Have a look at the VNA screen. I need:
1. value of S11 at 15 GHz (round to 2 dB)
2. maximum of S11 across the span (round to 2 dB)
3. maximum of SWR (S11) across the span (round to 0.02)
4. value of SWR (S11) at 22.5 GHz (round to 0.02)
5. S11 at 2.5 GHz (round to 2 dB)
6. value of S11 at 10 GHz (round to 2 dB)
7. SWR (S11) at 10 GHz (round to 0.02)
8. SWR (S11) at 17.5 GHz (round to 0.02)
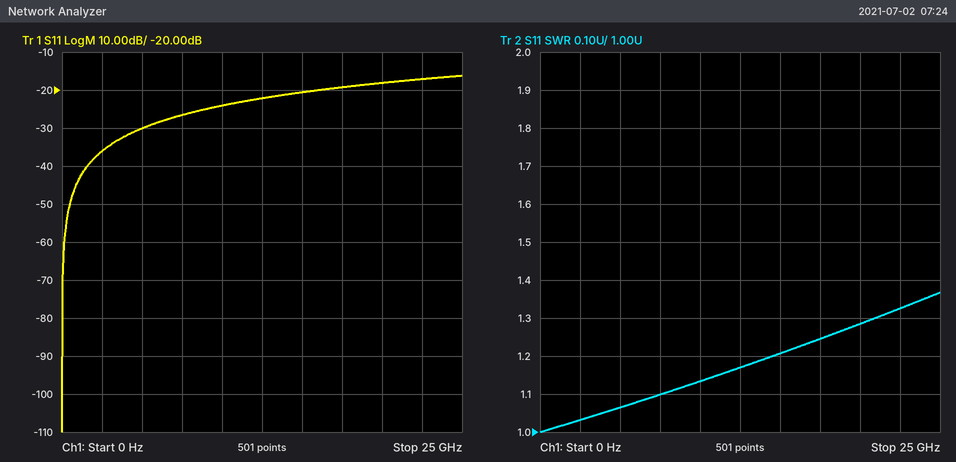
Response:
-20 dB
-16 dB
1.36
1.32
-36 dB
-24 dB
1.14
1.24
